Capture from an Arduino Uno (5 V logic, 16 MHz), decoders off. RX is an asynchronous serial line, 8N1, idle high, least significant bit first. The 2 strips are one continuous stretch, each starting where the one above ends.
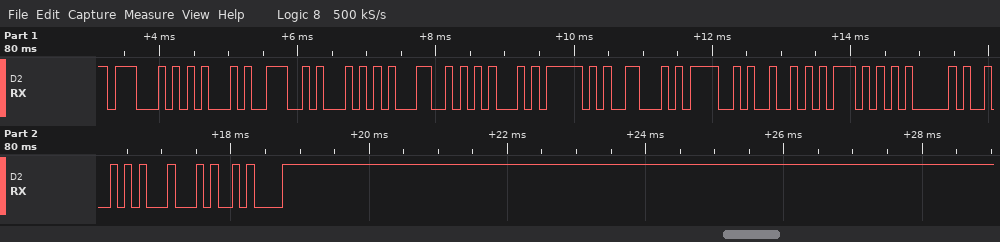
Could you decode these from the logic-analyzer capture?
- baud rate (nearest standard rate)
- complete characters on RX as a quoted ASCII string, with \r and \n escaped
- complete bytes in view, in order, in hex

9600 baud
"GENTLE_FORWARD\n"
47 45 4E 54 4C 45 5F 46 4F 52 57 41 52 44 0A
